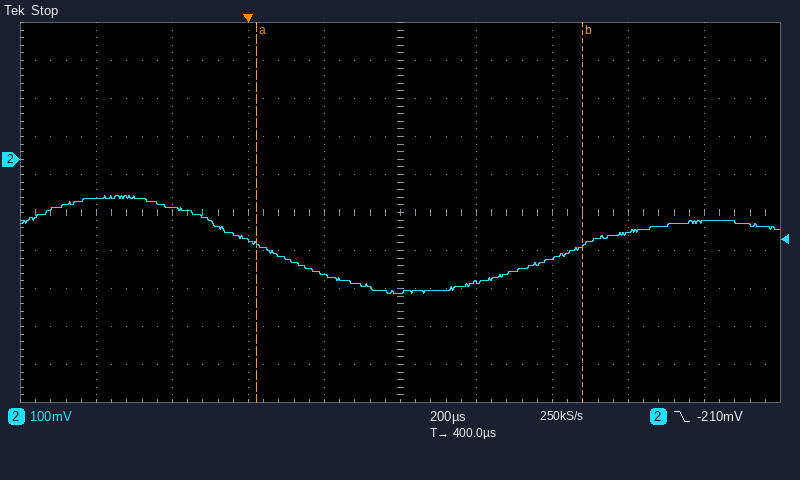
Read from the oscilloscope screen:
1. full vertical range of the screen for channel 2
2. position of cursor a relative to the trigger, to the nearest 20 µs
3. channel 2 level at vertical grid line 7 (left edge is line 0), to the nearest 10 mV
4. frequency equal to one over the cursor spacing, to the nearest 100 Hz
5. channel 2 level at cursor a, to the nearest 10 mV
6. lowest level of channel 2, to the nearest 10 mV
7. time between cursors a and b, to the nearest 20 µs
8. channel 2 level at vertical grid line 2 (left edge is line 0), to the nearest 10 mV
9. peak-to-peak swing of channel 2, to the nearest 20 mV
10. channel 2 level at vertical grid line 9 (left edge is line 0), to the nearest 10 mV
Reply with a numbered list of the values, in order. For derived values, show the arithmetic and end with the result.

1. 1 V
2. +20 µs
3. -260 mV
4. 1 / 860 µs ≈ 1.2 kHz
5. -220 mV
6. -350 mV
7. 860 µs
8. -130 mV
9. 260 mV
10. -160 mV
